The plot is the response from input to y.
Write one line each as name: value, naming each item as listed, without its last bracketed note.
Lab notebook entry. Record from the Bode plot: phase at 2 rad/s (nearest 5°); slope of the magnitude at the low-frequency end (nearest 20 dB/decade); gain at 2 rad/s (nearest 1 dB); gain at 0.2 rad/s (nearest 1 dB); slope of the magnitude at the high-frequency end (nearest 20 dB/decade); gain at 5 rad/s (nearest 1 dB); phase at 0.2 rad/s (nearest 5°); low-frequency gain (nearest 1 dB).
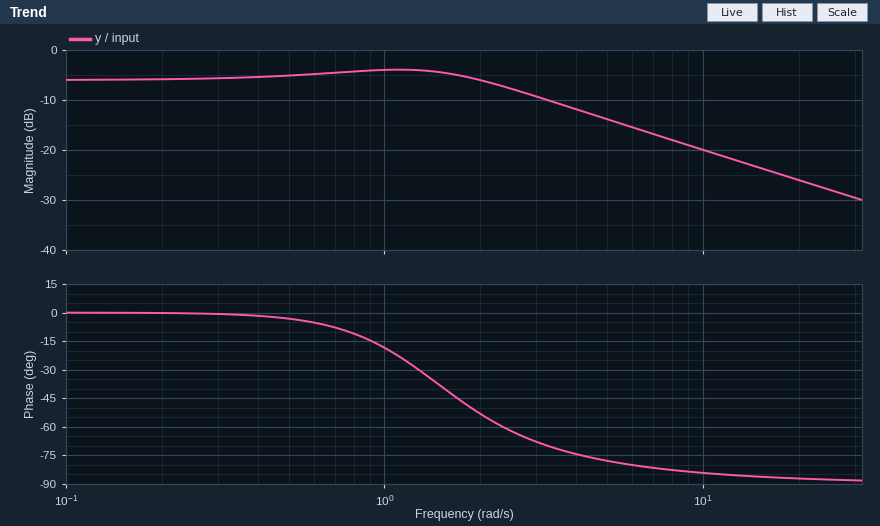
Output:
phase at 2 rad/s: -55°
slope of the magnitude at the low-frequency end: 0 dB/decade
gain at 2 rad/s: -6 dB
gain at 0.2 rad/s: -6 dB
slope of the magnitude at the high-frequency end: -20 dB/decade
gain at 5 rad/s: -14 dB
phase at 0.2 rad/s: 0°
low-frequency gain: -6 dB
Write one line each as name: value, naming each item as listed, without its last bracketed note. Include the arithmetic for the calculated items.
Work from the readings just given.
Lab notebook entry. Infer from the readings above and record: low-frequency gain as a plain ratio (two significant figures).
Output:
low-frequency gain as a plain ratio: 10^(-6 / 20) = 0.50
